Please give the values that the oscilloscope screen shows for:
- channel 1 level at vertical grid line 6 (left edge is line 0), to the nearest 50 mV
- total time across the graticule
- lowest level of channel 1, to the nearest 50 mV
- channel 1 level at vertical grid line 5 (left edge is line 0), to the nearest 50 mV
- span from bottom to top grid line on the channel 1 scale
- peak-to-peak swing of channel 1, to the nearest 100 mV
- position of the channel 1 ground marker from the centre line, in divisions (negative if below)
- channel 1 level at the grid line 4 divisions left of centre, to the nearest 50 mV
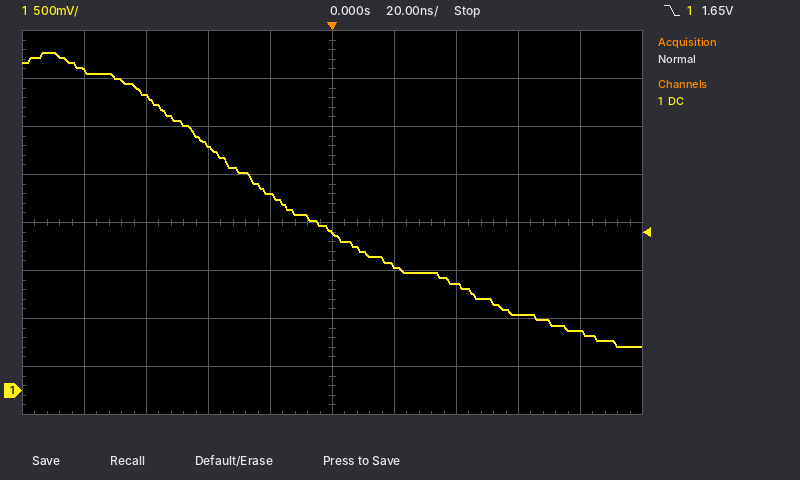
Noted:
1.30 V
200 ns
450 mV
1.65 V
4 V
3.10 V
-3.5 div
3.35 V
